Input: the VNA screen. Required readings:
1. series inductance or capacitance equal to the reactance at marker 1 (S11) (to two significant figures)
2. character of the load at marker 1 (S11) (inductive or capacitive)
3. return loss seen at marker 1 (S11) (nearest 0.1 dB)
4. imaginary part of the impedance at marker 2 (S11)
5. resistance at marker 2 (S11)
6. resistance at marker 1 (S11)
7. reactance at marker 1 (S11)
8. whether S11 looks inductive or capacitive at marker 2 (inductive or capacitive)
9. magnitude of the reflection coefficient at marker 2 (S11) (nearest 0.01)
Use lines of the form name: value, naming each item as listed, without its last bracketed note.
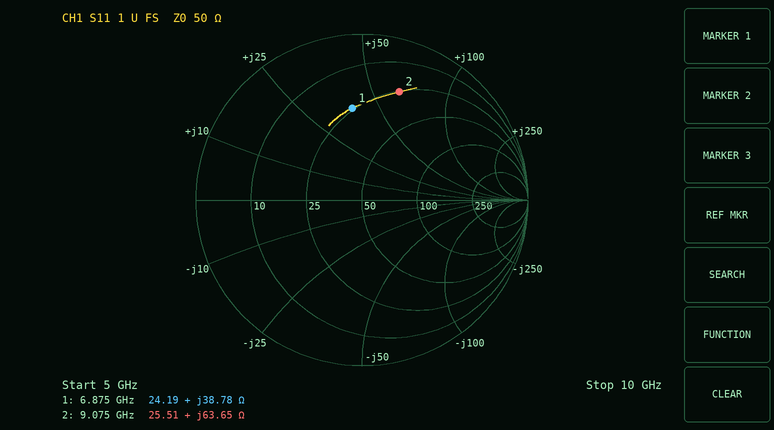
series inductance or capacitance equal to the reactance at marker 1 (S11): 900 pH
character of the load at marker 1 (S11): inductive
return loss seen at marker 1 (S11): 5.1 dB
imaginary part of the impedance at marker 2: +63.65 Ω
resistance at marker 2: 25.51 Ω
resistance at marker 1: 24.19 Ω
reactance at marker 1: +38.78 Ω
whether S11 looks inductive or capacitive at marker 2: inductive
magnitude of the reflection coefficient at marker 2 (S11): 0.69
